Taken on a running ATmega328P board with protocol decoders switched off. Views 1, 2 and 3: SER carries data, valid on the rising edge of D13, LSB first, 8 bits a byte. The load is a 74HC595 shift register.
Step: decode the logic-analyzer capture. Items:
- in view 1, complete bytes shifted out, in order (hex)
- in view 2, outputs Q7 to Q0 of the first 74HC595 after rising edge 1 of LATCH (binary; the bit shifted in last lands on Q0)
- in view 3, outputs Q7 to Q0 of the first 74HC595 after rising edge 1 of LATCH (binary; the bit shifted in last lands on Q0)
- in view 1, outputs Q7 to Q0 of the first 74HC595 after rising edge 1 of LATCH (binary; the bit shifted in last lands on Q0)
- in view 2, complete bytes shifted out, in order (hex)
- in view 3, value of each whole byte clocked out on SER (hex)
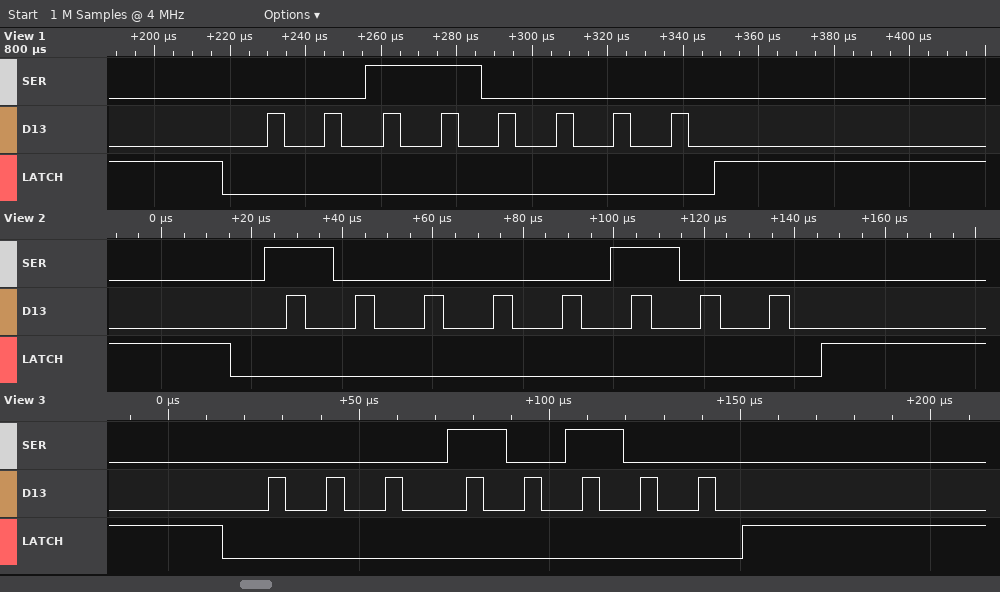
0C
10000100
00010100
00110000
21
0x28
